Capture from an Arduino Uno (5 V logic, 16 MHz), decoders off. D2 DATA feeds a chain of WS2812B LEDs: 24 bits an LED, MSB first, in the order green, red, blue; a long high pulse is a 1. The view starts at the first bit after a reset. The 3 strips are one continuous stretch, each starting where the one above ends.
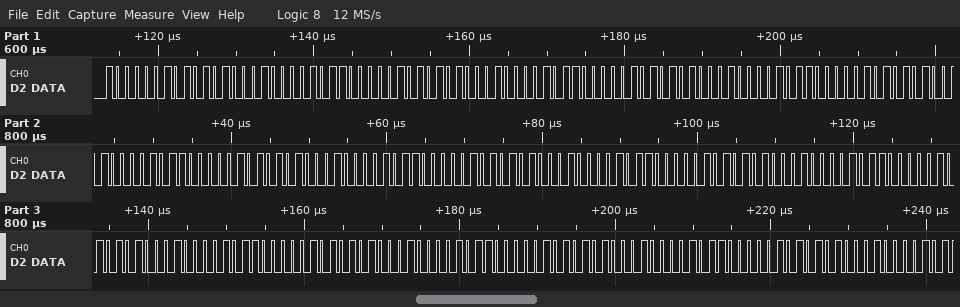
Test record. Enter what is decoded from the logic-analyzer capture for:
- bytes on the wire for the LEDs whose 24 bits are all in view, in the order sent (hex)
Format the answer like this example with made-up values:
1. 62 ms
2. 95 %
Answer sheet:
1. 82 A8 85 82 A8 85 82 A8 85 82 A8 85 82 A8 85 82 A8 85 82 A8 85 82 A8 85 82 A8 85 82 A8 85 82 A8 85
